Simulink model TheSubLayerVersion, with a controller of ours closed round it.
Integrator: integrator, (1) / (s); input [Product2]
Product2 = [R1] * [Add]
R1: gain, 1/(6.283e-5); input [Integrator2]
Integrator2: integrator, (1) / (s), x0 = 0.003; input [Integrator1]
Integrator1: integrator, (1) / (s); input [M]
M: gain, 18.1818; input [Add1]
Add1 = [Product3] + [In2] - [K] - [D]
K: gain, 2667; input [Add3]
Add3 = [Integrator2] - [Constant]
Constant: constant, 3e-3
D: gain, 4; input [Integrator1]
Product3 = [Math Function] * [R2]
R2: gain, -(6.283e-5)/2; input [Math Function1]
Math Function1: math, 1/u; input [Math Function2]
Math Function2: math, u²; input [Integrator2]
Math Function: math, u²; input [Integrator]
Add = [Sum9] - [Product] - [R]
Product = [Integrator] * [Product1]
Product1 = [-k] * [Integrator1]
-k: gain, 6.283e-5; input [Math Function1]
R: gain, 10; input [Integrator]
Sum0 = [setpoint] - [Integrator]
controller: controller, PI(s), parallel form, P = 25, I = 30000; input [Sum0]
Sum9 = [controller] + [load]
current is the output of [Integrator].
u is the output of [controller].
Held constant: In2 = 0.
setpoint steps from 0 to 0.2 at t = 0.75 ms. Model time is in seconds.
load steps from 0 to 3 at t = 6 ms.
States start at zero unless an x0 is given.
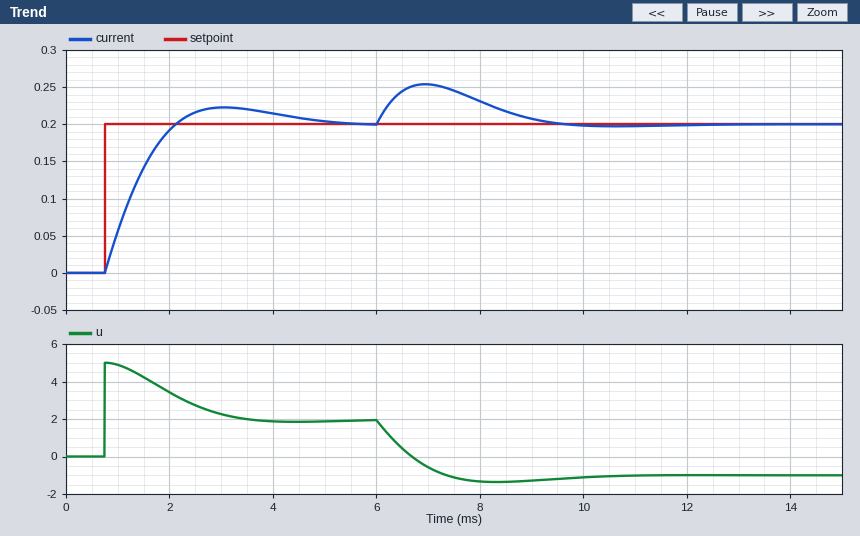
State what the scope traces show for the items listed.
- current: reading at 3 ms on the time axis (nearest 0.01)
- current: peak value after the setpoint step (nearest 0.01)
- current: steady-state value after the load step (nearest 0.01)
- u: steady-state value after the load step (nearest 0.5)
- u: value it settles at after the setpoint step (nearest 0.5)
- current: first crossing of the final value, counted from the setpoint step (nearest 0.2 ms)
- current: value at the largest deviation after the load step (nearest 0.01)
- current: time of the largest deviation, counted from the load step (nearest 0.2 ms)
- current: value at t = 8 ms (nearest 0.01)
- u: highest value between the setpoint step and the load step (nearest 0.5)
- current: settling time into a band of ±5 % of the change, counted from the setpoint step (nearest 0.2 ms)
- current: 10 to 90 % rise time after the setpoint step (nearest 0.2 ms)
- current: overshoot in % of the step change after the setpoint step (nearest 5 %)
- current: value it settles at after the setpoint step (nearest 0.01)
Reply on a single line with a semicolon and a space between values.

0.22; 0.22; 0.20; -1.0; 2.0; 1.4 ms; 0.25; 1.0 ms; 0.23; 5.0; 3.6 ms; 1.0 ms; 10 %; 0.20
